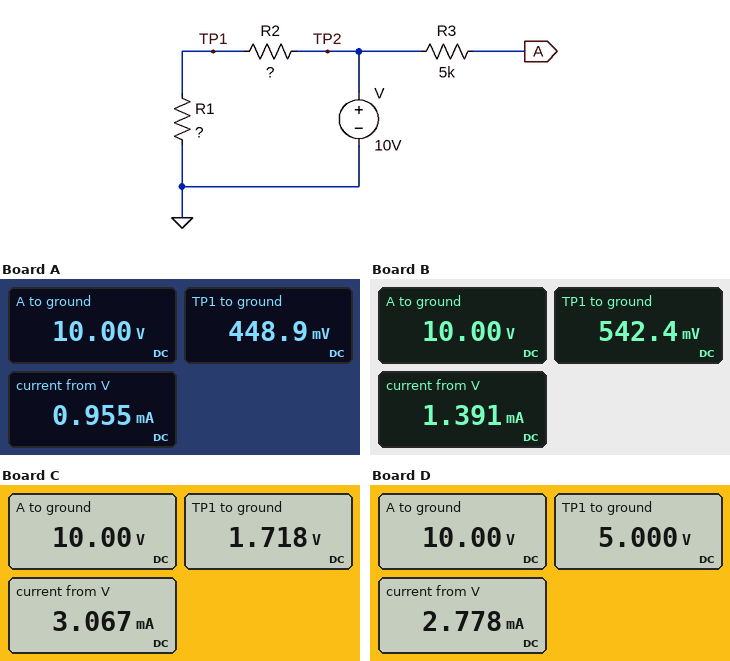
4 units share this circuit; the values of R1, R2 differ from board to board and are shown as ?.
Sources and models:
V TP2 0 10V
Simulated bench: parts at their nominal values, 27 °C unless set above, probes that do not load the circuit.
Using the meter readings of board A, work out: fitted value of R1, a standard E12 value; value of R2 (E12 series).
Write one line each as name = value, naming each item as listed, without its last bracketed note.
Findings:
fitted value of R1, a standard E12 value = 470 Ω
value of R2 = 10 kΩ
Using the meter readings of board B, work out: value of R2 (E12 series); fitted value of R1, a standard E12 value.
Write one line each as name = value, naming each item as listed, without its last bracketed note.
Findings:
value of R2 = 6.8 kΩ
fitted value of R1, a standard E12 value = 390 Ω
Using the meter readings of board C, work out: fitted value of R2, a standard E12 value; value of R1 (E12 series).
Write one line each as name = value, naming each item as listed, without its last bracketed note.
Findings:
fitted value of R2, a standard E12 value = 2.7 kΩ
value of R1 = 560 Ω
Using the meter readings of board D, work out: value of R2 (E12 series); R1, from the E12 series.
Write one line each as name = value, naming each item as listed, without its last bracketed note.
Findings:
value of R2 = 1.8 kΩ
R1, from the E12 series = 1.8 kΩ
